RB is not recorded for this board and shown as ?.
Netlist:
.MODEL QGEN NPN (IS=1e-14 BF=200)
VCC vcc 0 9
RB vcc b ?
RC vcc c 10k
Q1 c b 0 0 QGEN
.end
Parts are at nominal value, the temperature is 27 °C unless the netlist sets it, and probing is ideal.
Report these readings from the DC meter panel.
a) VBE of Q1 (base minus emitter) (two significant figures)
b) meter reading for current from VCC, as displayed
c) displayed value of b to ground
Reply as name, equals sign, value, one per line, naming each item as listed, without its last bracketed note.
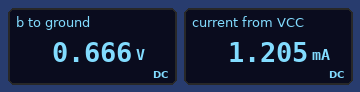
VBE of Q1 (base minus emitter) = 670 mV
meter reading for current from VCC, as displayed = 1.205 mA
displayed value of b to ground = 0.666 V
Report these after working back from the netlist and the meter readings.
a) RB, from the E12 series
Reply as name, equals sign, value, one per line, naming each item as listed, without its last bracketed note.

RB, from the E12 series = 27 kΩ
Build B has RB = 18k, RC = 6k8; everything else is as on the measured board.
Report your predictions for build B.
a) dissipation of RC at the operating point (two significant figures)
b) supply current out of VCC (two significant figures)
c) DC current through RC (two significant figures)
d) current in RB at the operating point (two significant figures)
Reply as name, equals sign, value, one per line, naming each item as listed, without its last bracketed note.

dissipation of RC at the operating point = 12 mW
supply current out of VCC = 1.8 mA
DC current through RC = 1.3 mA
current in RB at the operating point = 460 µA
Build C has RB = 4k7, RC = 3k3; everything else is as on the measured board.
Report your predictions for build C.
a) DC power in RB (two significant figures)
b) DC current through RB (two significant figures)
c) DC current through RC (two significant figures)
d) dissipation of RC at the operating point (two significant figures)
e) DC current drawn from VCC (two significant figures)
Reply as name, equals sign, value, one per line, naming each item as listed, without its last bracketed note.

DC power in RB = 15 mW
DC current through RB = 1.8 mA
DC current through RC = 2.7 mA
dissipation of RC at the operating point = 24 mW
DC current drawn from VCC = 4.5 mA
